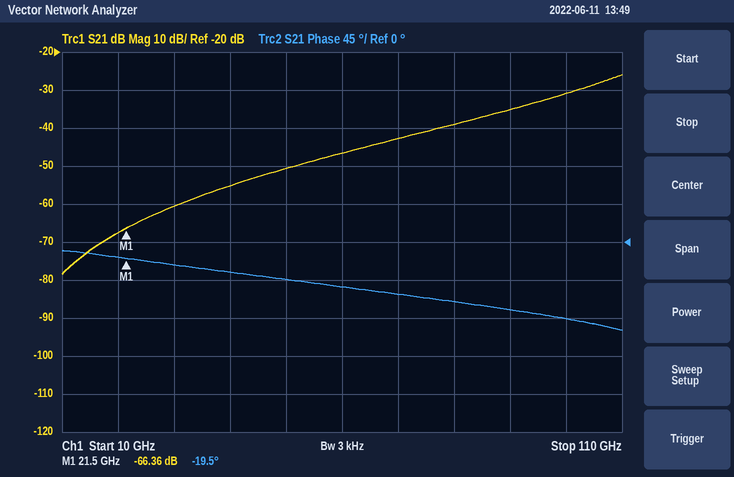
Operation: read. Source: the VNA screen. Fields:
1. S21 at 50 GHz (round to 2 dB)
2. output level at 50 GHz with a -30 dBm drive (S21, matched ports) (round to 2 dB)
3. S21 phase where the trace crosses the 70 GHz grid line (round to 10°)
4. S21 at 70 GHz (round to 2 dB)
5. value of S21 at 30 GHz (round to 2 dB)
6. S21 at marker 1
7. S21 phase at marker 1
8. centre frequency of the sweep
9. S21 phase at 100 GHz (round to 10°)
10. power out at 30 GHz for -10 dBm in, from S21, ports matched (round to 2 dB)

-50 dB
-80 dBm
-60°
-42 dB
-60 dB
-66.36 dB
-19.5°
60 GHz
-90°
-70 dBm
